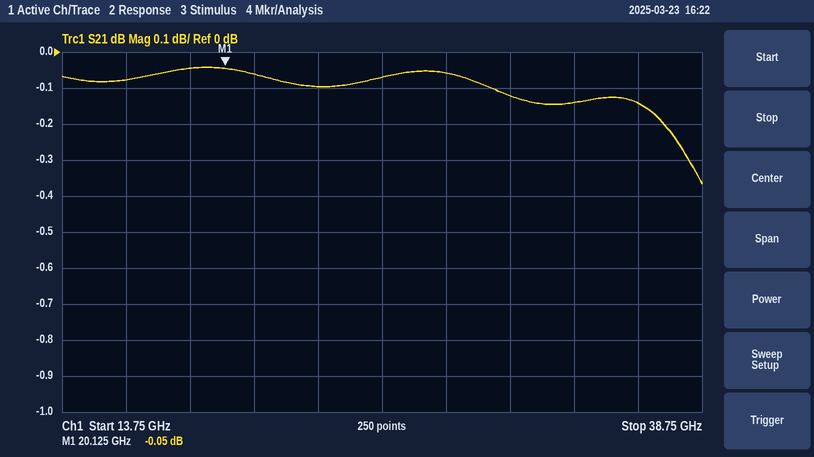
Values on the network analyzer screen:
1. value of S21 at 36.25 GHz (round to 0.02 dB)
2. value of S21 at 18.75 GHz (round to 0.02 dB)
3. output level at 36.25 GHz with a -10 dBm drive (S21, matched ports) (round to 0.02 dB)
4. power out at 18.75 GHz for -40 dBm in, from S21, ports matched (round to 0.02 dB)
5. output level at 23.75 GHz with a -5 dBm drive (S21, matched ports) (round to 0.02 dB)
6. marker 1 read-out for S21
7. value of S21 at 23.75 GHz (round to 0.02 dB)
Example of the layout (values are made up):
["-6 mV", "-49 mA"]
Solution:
["-0.14 dB", "-0.04 dB", "-10.14 dBm", "-40.04 dBm", "-5.10 dBm", "-0.05 dB", "-0.10 dB"]
